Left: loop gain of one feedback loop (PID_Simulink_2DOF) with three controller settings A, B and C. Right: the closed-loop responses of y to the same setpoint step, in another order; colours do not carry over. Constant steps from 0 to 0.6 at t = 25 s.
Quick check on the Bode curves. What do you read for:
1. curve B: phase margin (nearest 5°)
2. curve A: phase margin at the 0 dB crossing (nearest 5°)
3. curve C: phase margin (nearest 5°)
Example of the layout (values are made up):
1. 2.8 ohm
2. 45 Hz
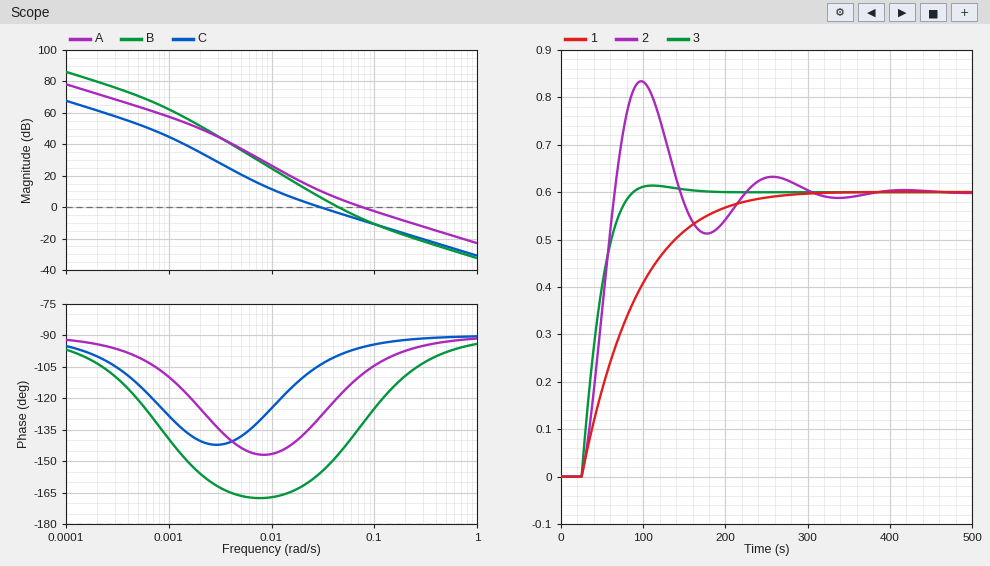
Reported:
1. 35°
2. 70°
3. 75°
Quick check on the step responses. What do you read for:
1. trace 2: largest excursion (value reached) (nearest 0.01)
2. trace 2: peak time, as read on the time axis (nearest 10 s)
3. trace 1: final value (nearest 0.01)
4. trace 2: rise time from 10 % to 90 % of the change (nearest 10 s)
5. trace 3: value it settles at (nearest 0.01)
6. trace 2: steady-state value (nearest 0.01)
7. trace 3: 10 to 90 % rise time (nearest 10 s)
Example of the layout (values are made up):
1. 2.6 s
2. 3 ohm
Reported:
1. 0.83
2. 100 s
3. 0.60
4. 30 s
5. 0.60
6. 0.60
7. 40 s
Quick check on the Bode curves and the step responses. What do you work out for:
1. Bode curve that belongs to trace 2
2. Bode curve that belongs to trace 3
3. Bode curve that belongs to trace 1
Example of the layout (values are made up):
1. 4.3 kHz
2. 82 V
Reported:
1. B
2. A
3. C
